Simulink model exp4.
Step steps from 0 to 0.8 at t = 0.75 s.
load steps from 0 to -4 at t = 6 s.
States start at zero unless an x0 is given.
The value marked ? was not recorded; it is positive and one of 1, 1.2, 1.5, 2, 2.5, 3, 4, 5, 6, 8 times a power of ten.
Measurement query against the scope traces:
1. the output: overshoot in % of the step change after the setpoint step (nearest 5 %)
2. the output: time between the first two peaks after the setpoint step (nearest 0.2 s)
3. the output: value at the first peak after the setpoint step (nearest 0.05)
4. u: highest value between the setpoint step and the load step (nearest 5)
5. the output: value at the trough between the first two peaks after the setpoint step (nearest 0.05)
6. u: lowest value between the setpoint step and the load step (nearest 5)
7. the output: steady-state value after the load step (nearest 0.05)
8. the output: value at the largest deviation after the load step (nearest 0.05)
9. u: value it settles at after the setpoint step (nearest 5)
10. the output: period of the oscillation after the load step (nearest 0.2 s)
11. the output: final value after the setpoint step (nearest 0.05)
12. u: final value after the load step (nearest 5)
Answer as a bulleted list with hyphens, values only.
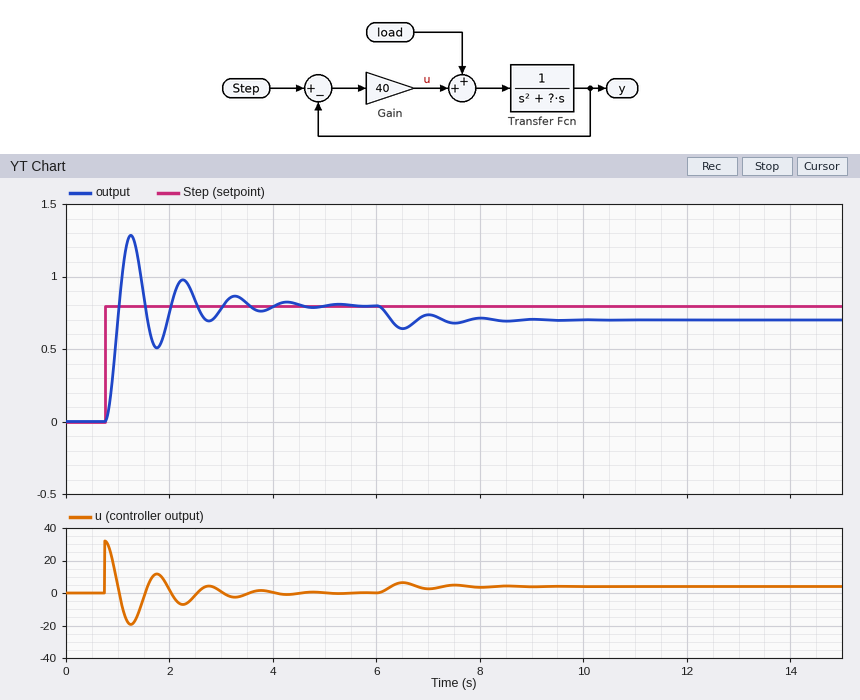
- 60 %
- 1.0 s
- 1.30
- 30
- 0.50
- -20
- 0.70
- 0.65
- 0
- 1.0 s
- 0.80
- 5
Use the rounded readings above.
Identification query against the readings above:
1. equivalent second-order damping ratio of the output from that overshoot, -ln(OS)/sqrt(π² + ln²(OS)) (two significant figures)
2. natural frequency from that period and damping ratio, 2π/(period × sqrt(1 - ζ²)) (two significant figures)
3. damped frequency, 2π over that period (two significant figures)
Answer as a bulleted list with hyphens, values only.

- 0.16
- 6.4 rad/s
- 6.3 rad/s
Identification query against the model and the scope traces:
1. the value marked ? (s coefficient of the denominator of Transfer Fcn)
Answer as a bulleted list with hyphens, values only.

- 2
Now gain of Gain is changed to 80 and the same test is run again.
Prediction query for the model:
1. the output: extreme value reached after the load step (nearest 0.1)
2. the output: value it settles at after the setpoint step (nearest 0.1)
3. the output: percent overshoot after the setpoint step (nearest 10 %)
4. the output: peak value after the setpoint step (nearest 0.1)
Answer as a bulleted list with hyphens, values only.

- 0.7
- 0.8
- 70 %
- 1.4
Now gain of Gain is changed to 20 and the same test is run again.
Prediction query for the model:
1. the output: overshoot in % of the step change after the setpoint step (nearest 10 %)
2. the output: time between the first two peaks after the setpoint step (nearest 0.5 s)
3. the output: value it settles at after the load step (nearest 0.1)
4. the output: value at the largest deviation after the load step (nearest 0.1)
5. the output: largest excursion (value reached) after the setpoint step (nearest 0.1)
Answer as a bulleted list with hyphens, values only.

- 50 %
- 1.5 s
- 0.6
- 0.5
- 1.2
